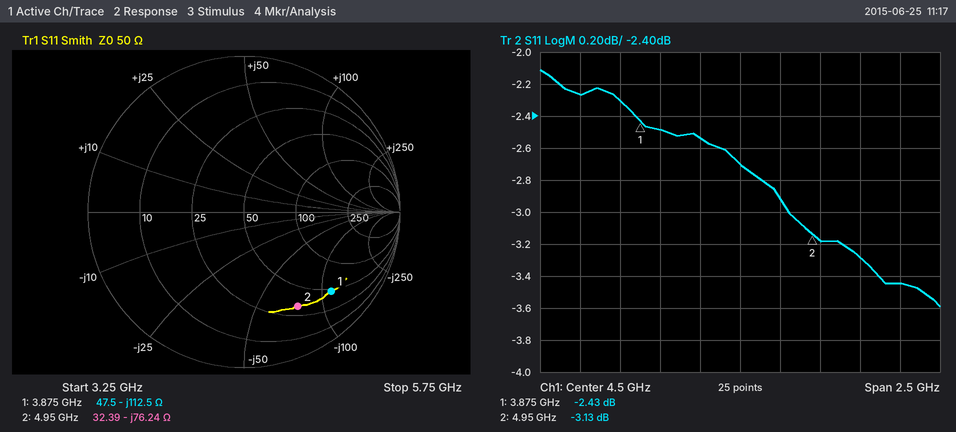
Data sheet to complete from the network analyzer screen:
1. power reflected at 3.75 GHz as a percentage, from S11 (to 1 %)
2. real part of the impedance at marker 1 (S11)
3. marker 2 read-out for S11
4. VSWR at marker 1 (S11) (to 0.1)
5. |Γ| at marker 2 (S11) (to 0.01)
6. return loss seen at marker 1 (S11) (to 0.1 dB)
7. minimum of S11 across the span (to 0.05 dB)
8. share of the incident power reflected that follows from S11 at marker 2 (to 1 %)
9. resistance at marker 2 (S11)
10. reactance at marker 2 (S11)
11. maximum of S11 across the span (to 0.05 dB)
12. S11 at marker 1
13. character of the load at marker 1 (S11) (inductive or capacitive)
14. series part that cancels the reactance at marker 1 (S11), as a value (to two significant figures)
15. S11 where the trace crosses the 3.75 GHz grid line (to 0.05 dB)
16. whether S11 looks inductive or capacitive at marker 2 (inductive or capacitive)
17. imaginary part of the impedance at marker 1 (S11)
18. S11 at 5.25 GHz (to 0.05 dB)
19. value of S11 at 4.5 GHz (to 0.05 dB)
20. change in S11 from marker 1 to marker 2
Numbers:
59 %
47.5 Ω
-3.13 dB
7.2
0.70
2.4 dB
-3.60 dB
49 %
32.39 Ω
-76.24 Ω
-2.10 dB
-2.43 dB
capacitive
4.6 nH
-2.30 dB
capacitive
-112.5 Ω
-3.30 dB
-2.70 dB
-0.70 dB
